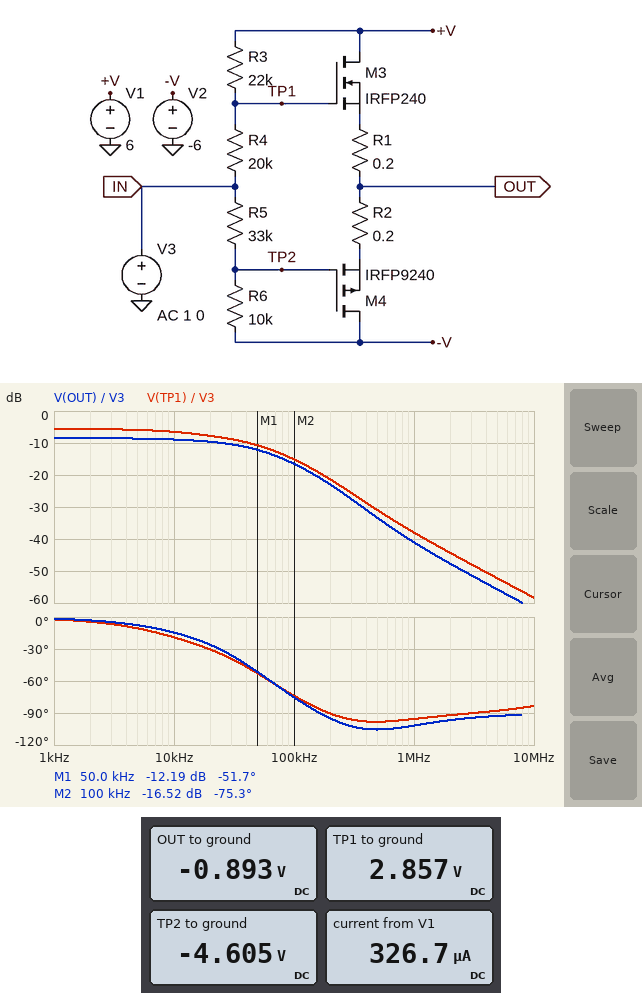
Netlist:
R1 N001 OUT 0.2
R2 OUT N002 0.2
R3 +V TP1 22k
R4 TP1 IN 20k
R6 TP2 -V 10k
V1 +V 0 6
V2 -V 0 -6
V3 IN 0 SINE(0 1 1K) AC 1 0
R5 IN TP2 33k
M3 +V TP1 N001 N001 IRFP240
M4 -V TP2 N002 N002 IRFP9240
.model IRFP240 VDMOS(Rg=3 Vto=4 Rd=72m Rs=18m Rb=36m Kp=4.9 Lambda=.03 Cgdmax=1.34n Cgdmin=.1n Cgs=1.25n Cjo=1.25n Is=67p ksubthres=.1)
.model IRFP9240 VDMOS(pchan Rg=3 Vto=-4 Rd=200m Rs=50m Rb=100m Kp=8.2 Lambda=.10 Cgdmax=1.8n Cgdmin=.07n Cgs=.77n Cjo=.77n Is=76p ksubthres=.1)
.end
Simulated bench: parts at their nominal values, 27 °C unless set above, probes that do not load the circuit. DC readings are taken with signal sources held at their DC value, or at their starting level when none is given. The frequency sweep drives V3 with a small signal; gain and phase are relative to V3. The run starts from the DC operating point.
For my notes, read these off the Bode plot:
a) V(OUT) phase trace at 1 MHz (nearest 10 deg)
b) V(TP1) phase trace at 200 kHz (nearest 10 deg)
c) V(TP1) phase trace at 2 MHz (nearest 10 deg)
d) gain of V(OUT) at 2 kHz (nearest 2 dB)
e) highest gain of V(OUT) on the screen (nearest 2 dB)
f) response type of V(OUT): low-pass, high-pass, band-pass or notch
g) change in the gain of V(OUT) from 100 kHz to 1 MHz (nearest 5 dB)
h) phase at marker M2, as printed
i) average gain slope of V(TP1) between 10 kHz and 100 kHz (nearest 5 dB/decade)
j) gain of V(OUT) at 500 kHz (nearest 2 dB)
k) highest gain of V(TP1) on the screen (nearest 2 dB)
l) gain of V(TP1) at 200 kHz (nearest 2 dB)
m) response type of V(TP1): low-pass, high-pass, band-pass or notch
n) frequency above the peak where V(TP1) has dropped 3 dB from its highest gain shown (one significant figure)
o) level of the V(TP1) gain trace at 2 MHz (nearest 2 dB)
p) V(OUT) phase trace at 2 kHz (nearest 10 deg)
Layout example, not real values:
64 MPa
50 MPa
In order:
-100 deg
-90 deg
-90 deg
-8 dB
-8 dB
low-pass
-25 dB
-75.3 deg
-10 dB/decade
-34 dB
-6 dB
-22 dB
low-pass
30 kHz
-44 dB
0 deg
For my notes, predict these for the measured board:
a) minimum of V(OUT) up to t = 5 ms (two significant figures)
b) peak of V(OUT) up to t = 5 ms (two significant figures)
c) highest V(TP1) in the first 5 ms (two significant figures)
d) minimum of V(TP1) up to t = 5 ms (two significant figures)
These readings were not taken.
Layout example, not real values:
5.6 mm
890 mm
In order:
-1.3 V
-520 mV
3.4 V
2.3 V
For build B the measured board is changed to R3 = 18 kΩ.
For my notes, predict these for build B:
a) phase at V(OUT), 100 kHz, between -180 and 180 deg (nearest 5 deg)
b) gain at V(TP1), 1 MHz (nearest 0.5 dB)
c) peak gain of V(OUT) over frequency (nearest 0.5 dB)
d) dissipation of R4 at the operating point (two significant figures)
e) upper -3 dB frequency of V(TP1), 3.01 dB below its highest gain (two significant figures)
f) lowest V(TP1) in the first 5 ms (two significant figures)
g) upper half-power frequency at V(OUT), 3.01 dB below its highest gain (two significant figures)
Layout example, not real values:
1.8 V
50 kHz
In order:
-65 deg
-35.0 dB
-9.0 dB
500 µW
31 kHz
2.7 V
43 kHz
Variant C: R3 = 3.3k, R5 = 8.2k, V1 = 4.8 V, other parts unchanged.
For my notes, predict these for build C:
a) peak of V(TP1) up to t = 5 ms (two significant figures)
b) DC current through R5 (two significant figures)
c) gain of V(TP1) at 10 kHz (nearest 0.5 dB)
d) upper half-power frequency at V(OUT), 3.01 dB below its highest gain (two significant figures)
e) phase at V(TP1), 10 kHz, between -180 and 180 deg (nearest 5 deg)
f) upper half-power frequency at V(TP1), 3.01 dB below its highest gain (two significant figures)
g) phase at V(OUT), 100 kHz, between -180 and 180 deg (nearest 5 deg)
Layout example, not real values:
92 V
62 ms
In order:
4.3 V
330 µA
-16.5 dB
1.7 kHz
0 deg
100 kHz
-55 deg
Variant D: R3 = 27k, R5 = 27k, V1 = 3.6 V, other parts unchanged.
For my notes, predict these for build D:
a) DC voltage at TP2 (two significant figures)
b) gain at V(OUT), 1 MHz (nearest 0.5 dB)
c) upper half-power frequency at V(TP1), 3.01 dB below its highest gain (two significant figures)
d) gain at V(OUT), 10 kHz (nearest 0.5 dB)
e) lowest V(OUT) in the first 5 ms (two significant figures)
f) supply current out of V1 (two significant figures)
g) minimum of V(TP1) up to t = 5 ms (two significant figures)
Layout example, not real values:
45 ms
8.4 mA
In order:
-4.4 V
-42.0 dB
16 kHz
-10.5 dB
-1.8 V
77 µA
960 mV
